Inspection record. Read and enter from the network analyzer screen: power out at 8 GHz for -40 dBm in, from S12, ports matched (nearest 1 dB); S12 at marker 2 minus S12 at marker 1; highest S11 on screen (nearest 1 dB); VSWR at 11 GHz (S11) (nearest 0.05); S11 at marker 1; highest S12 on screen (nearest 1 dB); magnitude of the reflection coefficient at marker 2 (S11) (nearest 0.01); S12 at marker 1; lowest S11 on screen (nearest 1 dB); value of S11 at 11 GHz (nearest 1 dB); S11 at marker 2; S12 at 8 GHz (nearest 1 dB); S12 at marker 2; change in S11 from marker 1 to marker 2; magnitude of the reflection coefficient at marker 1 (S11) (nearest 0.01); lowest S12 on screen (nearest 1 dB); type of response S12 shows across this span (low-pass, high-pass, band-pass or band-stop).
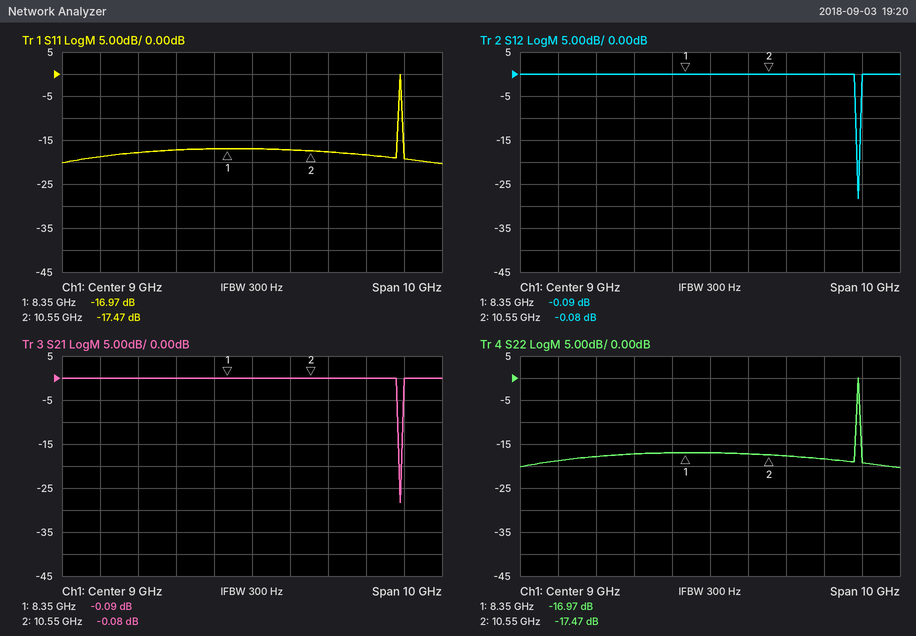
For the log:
-40 dBm
0.01 dB
0 dB
1.30
-16.97 dB
0 dB
0.13
-0.09 dB
-20 dB
-18 dB
-17.47 dB
0 dB
-0.08 dB
-0.50 dB
0.14
-28 dB
band-stop
